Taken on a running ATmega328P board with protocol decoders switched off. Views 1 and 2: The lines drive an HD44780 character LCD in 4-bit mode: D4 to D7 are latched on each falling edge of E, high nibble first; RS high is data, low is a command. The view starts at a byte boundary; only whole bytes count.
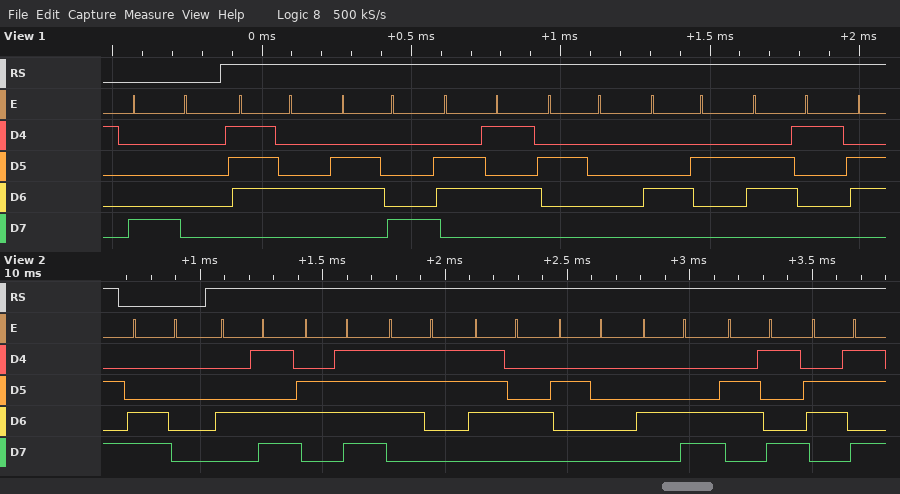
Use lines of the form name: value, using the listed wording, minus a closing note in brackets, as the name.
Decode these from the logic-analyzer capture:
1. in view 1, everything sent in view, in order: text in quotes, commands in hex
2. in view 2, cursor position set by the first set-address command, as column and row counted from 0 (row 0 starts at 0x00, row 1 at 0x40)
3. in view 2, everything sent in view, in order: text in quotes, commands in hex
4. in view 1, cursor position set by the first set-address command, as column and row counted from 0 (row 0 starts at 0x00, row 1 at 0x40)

in view 1, everything sent in view, in order: text in quotes, commands in hex: 0x80 "the Ba"
in view 2, cursor position set by the first set-address command, as column and row counted from 0: column 0, row 1
in view 2, everything sent in view, in order: text in quotes, commands in hex: 0xC0 "Most Lik"
in view 1, cursor position set by the first set-address command, as column and row counted from 0: column 0, row 0
